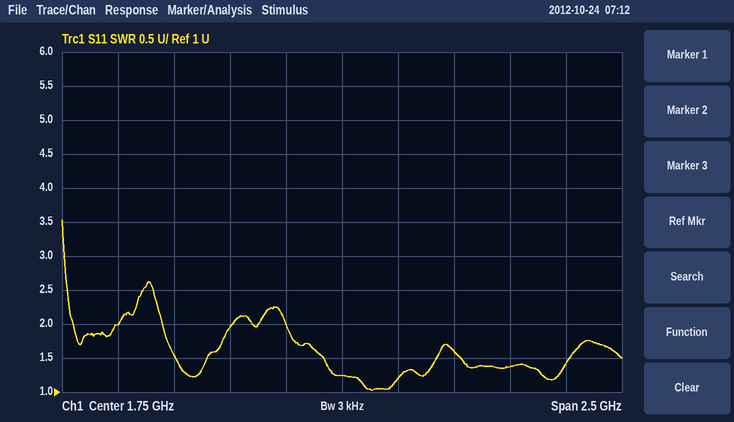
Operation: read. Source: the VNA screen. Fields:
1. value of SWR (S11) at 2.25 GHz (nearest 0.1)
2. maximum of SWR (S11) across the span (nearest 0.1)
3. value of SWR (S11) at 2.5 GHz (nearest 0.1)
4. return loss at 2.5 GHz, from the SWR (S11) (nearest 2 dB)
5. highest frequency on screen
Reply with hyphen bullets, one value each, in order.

- 1.6
- 3.5
- 1.4
- 16 dB
- 3 GHz
